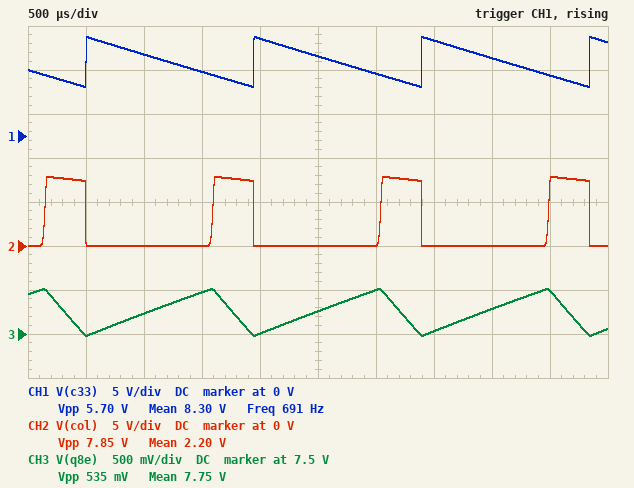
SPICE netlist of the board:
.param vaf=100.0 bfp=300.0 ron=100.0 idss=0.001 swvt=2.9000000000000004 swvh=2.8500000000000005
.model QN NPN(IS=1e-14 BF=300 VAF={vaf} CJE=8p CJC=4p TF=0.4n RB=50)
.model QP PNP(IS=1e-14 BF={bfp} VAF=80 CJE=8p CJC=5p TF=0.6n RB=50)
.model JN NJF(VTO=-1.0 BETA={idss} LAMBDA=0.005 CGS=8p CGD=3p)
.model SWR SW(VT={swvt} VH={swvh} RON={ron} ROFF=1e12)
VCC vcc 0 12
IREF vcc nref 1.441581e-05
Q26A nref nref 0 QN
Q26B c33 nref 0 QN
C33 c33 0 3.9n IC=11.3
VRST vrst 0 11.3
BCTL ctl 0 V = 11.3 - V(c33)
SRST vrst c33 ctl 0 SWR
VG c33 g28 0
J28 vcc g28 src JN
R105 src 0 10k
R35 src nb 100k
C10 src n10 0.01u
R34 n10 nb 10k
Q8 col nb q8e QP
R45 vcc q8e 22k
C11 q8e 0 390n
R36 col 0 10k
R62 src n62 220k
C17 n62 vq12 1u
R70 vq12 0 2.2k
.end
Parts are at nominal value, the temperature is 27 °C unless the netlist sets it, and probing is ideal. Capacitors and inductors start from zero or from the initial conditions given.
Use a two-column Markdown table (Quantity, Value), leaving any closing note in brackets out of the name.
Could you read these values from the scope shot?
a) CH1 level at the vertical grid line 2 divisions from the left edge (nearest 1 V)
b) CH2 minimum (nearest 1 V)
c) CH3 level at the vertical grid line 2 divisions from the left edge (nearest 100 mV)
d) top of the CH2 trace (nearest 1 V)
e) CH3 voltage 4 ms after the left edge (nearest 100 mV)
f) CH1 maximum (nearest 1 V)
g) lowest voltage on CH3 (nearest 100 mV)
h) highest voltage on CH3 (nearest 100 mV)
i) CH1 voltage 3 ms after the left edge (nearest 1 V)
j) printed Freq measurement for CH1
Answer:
| Quantity | Value |
|---|---|
| CH1 level at the vertical grid line 2 divisions from the left edge | 9 V |
| CH2 minimum | 0 V |
| CH3 level at the vertical grid line 2 divisions from the left edge | 7.7 V |
| top of the CH2 trace | 8 V |
| CH3 voltage 4 ms after the left edge | 7.8 V |
| CH1 maximum | 11 V |
| lowest voltage on CH3 | 7.5 V |
| highest voltage on CH3 | 8.0 V |
| CH1 voltage 3 ms after the left edge | 7 V |
| printed Freq measurement for CH1 | 691 Hz |
